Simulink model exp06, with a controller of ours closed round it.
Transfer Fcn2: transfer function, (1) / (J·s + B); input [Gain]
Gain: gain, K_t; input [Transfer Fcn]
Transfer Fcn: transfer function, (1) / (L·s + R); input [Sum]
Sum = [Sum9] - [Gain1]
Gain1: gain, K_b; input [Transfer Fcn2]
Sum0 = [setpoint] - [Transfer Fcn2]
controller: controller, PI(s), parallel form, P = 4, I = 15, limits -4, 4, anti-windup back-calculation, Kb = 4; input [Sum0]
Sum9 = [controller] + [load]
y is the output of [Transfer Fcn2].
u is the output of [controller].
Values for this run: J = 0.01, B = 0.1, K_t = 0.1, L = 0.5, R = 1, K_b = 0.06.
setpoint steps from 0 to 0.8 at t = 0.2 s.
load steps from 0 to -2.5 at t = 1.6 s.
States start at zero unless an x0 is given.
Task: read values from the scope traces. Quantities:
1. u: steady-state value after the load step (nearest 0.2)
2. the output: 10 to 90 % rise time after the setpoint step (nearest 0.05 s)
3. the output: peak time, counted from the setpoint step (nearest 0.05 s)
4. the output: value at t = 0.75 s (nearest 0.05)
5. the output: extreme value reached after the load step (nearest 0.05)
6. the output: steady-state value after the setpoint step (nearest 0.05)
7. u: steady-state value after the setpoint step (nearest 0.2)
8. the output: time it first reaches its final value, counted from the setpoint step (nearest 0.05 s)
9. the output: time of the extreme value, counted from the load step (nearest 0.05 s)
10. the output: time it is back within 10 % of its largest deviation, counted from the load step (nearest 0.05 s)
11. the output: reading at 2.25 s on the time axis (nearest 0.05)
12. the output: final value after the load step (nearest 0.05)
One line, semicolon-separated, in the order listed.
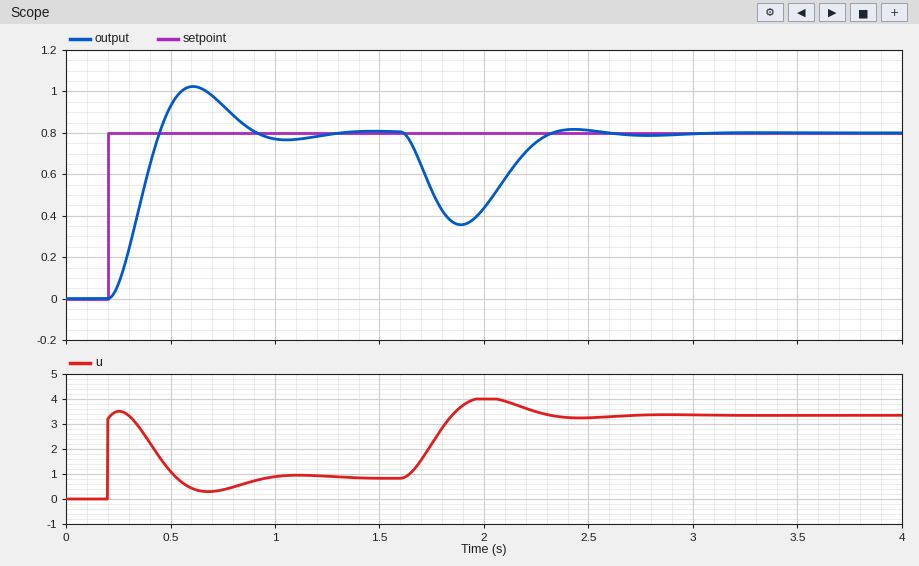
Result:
3.4; 0.15 s; 0.40 s; 0.95; 0.35; 0.80; 0.8; 0.25 s; 0.30 s; 0.65 s; 0.75; 0.80
